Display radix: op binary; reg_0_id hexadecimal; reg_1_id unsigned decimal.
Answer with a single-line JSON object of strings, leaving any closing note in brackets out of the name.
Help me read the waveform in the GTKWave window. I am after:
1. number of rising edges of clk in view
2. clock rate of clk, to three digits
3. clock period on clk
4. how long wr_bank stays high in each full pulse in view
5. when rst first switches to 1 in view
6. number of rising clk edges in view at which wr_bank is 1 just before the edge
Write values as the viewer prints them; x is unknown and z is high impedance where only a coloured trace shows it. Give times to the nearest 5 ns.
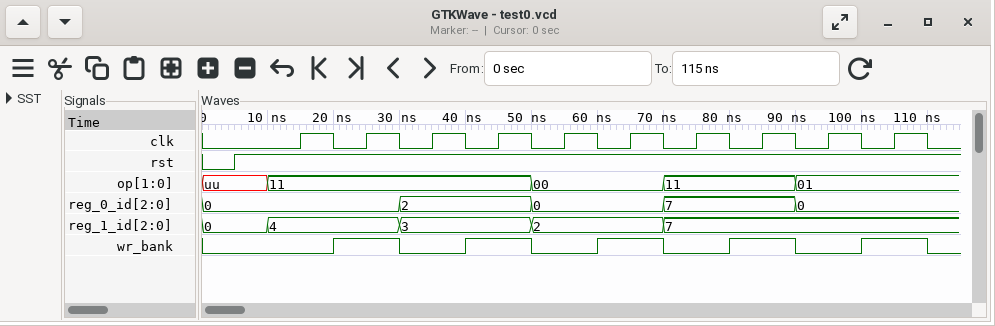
{"number of rising edges of clk in view": "10", "clock rate of clk, to three digits": "100 MHz", "clock period on clk": "10 ns", "how long wr_bank stays high in each full pulse in view": "10 ns, 10 ns, 10 ns, 10 ns, 10 ns", "when rst first switches to 1 in view": "5 ns", "number of rising clk edges in view at which wr_bank is 1 just before the edge": "5"}
